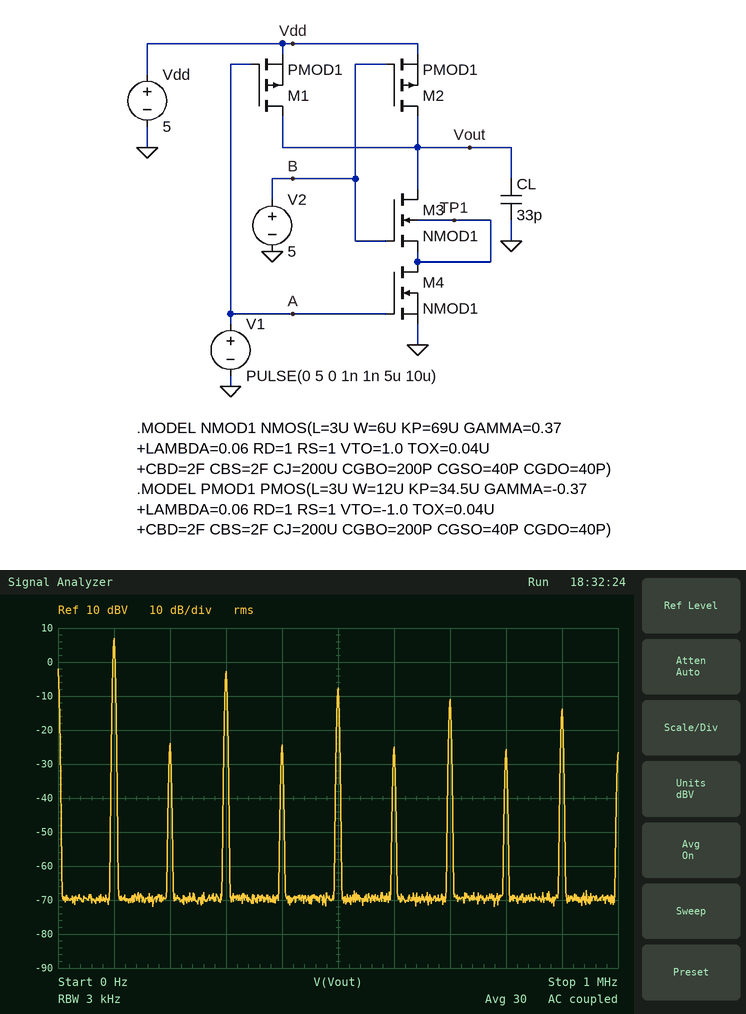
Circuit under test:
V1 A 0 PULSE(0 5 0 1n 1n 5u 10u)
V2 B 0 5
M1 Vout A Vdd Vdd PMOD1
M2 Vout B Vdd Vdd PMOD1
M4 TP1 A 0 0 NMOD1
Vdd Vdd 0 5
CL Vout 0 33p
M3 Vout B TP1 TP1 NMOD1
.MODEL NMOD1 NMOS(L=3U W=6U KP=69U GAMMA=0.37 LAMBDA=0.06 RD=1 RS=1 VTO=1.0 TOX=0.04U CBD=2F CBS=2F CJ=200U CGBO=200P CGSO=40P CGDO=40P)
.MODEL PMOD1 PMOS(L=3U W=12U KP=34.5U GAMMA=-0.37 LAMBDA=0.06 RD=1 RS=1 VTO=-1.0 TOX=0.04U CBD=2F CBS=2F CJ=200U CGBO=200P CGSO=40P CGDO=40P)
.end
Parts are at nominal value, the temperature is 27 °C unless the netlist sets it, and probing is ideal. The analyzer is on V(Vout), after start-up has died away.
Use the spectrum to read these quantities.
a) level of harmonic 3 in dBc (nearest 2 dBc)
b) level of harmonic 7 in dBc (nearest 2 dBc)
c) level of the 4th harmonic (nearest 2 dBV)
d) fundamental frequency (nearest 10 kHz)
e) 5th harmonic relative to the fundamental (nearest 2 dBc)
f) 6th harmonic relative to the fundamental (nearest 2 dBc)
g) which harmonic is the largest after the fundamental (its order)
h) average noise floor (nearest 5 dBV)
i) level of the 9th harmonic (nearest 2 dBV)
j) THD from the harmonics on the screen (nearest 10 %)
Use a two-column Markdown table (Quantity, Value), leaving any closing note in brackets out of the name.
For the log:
| Quantity | Value |
|---|---|
| level of harmonic 3 in dBc | -10 dBc |
| level of harmonic 7 in dBc | -18 dBc |
| level of the 4th harmonic | -24 dBV |
| fundamental frequency | 100 kHz |
| 5th harmonic relative to the fundamental | -14 dBc |
| 6th harmonic relative to the fundamental | -32 dBc |
| which harmonic is the largest after the fundamental | 3 |
| average noise floor | -70 dBV |
| level of the 9th harmonic | -14 dBV |
| THD from the harmonics on the screen | 40 % |
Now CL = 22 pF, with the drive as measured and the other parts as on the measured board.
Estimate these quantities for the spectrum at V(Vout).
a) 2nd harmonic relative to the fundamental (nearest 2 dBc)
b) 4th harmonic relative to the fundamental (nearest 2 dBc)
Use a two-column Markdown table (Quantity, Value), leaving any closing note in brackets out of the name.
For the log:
| Quantity | Value |
|---|---|
| 2nd harmonic relative to the fundamental | -34 dBc |
| 4th harmonic relative to the fundamental | -34 dBc |
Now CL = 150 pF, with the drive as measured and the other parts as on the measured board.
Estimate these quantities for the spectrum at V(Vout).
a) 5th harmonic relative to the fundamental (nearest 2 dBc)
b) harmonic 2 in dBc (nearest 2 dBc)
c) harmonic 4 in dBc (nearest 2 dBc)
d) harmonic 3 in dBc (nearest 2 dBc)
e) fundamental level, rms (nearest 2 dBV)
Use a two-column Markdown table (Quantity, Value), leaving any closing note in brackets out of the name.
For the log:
| Quantity | Value |
|---|---|
| 5th harmonic relative to the fundamental | -20 dBc |
| harmonic 2 in dBc | -20 dBc |
| harmonic 4 in dBc | -24 dBc |
| harmonic 3 in dBc | -12 dBc |
| fundamental level, rms | 6 dBV |
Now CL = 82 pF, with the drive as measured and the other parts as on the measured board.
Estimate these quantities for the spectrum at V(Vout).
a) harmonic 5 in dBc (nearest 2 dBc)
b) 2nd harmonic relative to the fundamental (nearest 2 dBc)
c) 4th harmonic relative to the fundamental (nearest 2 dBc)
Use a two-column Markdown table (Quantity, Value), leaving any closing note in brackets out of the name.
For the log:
| Quantity | Value |
|---|---|
| harmonic 5 in dBc | -16 dBc |
| 2nd harmonic relative to the fundamental | -24 dBc |
| 4th harmonic relative to the fundamental | -26 dBc |
